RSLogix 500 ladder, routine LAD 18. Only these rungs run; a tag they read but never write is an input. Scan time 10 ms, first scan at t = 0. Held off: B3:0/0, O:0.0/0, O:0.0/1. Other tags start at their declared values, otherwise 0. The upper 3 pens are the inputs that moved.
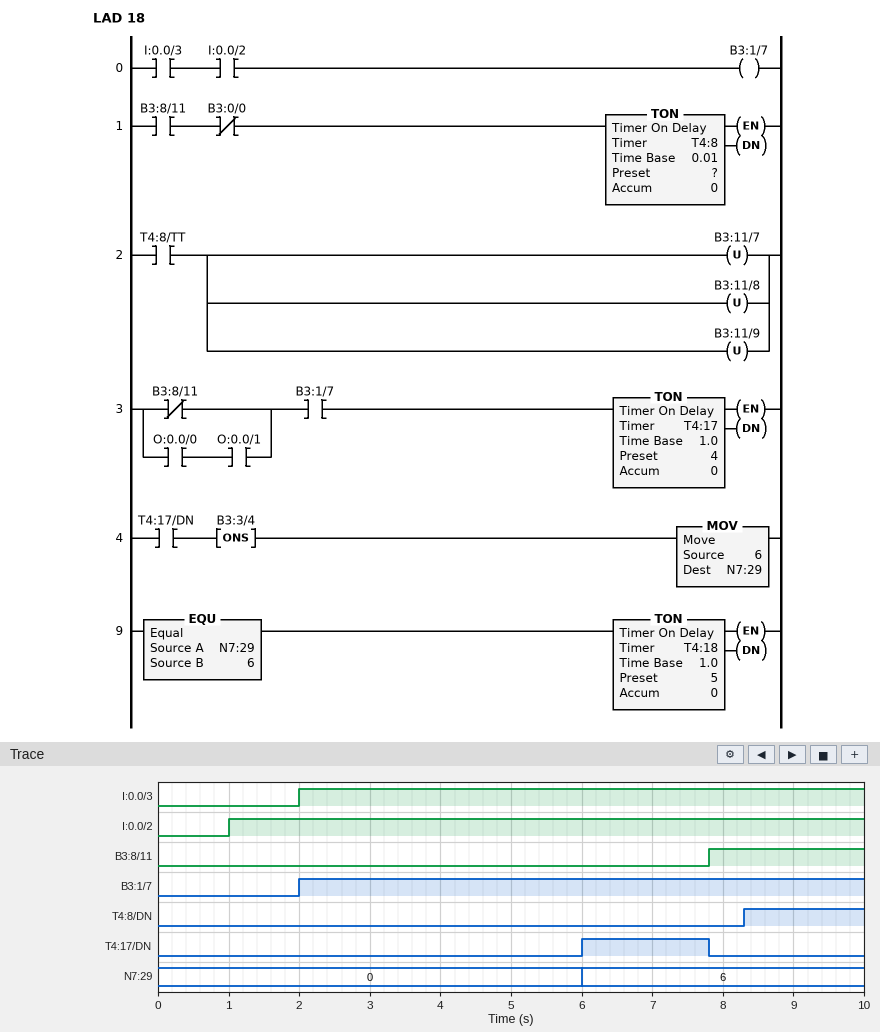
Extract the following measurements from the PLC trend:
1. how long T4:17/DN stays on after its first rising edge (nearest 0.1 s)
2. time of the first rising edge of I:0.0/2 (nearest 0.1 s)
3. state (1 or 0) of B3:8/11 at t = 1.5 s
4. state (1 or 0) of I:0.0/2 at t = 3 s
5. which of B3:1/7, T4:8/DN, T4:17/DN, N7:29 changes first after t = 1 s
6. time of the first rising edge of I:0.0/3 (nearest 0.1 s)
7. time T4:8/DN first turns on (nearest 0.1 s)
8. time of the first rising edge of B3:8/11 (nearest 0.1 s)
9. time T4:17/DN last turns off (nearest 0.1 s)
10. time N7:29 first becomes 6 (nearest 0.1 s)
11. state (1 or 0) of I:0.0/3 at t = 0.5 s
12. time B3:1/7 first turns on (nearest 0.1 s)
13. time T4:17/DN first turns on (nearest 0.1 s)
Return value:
1.8 s
1.0 s
0
1
B3:1/7
2.0 s
8.3 s
7.8 s
7.8 s
6.0 s
0
2.0 s
6.0 s
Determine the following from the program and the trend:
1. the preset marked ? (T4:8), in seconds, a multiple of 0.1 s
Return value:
0.5 s
